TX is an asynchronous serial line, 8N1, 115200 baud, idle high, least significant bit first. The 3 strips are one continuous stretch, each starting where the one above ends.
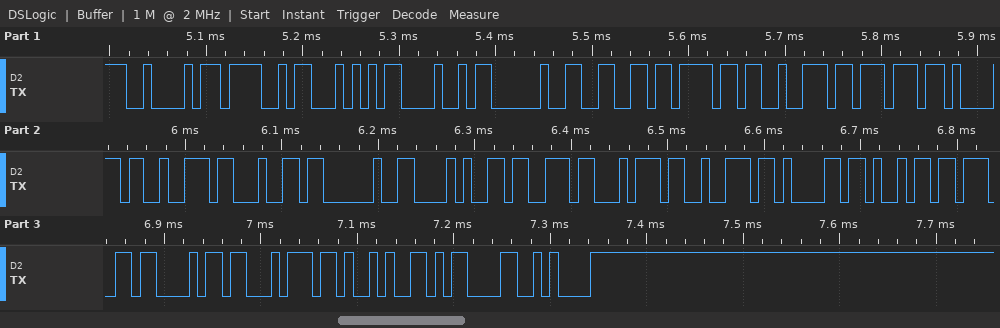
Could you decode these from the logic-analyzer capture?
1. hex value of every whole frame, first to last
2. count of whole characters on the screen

42 4F 54 48 20 66 6F 72 77 61 72 64 20 28 73 74 72 61 69 67 68 74 29 0D 0A
25
